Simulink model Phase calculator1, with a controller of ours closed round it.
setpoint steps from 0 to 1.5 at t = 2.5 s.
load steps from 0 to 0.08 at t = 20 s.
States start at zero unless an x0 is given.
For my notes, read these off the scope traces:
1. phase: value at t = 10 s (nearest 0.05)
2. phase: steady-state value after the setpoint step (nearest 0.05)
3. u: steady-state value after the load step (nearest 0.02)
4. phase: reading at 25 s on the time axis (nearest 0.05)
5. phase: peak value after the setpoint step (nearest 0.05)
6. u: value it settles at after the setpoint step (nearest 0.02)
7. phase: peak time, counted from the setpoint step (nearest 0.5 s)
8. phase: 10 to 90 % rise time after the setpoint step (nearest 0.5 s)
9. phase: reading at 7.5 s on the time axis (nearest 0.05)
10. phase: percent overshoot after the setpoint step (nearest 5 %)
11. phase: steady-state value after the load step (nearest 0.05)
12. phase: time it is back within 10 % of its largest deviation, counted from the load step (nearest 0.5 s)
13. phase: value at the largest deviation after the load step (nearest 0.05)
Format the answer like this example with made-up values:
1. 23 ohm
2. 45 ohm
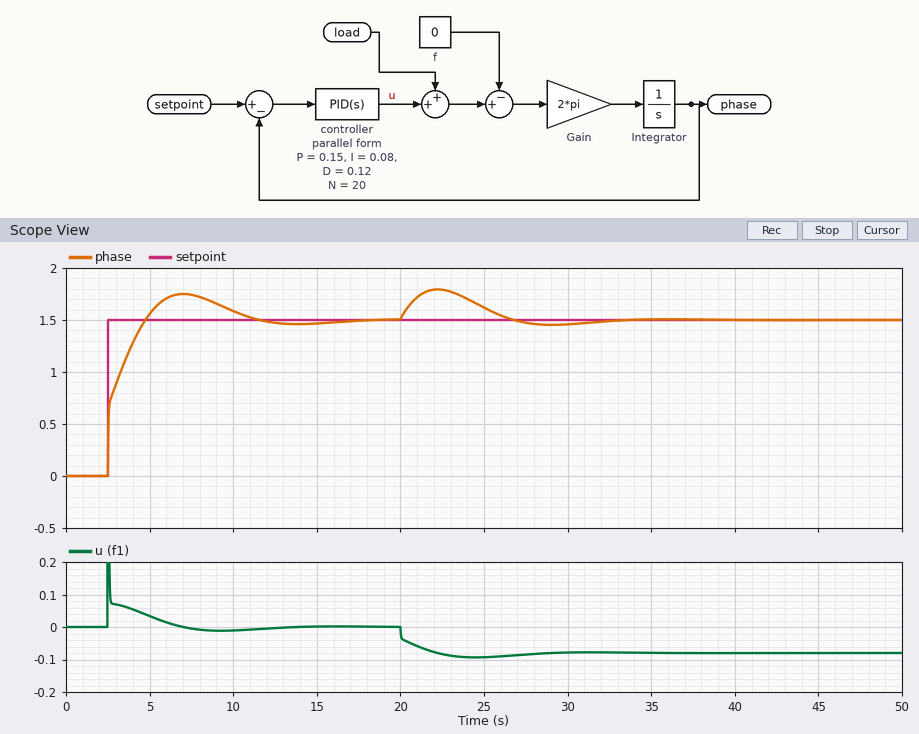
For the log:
1. 1.60
2. 1.50
3. -0.08
4. 1.60
5. 1.75
6. 0.00
7. 4.5 s
8. 1.5 s
9. 1.75
10. 15 %
11. 1.50
12. 11.0 s
13. 1.80
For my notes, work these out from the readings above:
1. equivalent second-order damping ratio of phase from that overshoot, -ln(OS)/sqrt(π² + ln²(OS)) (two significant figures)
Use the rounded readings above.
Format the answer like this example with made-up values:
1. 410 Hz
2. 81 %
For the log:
1. 0.52
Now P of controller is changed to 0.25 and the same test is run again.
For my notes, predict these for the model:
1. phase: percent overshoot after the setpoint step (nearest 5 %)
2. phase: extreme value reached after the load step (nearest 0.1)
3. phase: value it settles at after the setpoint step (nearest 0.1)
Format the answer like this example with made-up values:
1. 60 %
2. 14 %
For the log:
1. 10 %
2. 1.7
3. 1.5
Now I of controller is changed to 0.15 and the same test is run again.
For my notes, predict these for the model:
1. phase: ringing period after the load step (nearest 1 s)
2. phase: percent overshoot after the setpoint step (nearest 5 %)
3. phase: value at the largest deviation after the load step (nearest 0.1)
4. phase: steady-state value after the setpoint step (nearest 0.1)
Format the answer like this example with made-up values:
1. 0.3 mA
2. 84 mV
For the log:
1. 9 s
2. 20 %
3. 1.7
4. 1.5
